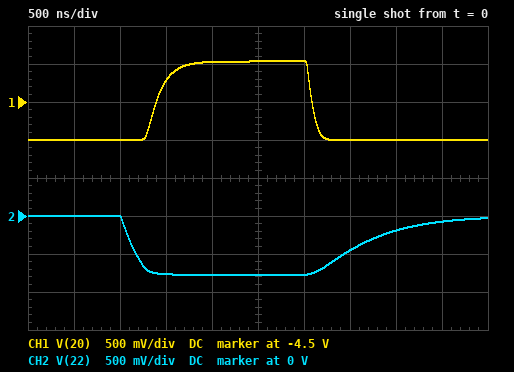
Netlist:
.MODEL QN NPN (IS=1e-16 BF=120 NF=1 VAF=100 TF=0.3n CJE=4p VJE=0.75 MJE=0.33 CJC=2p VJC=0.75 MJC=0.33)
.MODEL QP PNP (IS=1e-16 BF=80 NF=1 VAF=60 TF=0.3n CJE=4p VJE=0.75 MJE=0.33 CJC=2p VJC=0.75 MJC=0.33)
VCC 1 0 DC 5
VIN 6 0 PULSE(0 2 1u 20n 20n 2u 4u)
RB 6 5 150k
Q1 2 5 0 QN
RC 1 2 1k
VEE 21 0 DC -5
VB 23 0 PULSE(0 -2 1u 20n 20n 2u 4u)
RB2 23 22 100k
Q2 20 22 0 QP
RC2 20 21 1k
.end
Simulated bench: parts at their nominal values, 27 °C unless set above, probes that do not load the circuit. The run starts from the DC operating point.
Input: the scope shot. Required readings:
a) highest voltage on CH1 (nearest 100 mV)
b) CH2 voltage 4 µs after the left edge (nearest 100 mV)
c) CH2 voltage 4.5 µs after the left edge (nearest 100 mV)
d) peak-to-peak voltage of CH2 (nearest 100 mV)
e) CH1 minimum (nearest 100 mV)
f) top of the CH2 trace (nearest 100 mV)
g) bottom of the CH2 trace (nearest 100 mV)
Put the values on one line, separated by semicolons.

-4.0 V; -200 mV; -100 mV; 800 mV; -5.0 V; 0 V; -800 mV
